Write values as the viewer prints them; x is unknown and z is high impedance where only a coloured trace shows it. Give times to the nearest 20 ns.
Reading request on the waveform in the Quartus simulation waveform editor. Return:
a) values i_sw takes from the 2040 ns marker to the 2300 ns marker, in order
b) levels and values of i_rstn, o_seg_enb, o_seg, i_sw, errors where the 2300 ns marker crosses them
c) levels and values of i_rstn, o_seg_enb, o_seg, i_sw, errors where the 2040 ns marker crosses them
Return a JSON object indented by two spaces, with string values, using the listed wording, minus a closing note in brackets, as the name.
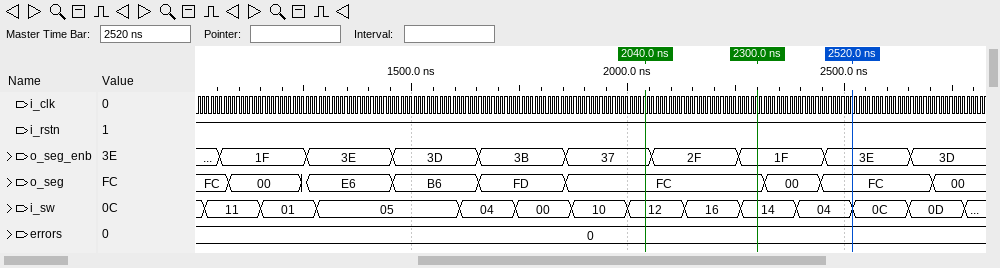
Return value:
{
  "values i_sw takes from the 2040 ns marker to the 2300 ns marker, in order": "12, 16, 14",
  "levels and values of i_rstn, o_seg_enb, o_seg, i_sw, errors where the 2300 ns marker crosses them": "i_rstn=1, o_seg_enb=1F, o_seg=FC, i_sw=14, errors=0",
  "levels and values of i_rstn, o_seg_enb, o_seg, i_sw, errors where the 2040 ns marker crosses them": "i_rstn=1, o_seg_enb=37, o_seg=FC, i_sw=12, errors=0"
}
